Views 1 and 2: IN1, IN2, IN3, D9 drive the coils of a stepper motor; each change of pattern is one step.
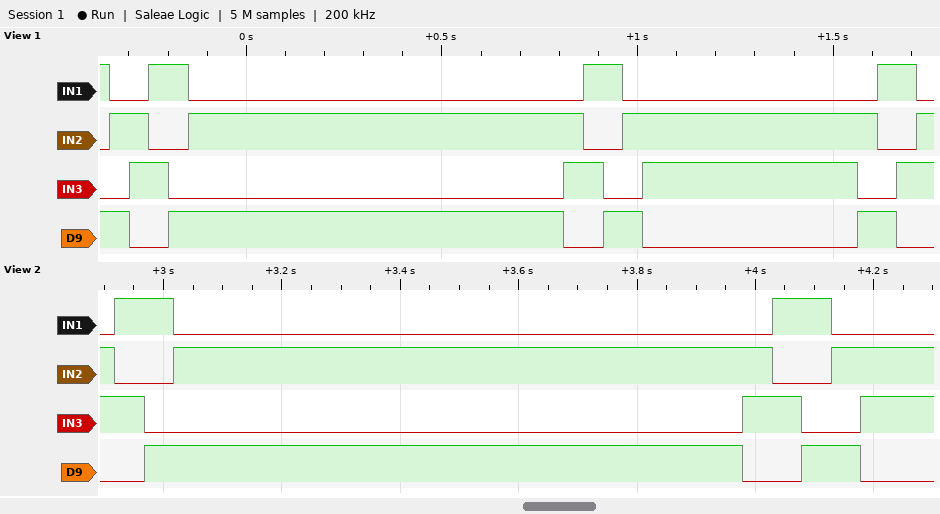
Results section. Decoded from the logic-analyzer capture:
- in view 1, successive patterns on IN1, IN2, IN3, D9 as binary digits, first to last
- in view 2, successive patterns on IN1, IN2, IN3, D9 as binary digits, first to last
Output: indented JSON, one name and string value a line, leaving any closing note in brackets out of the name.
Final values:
{
  "in view 1, successive patterns on IN1, IN2, IN3, D9 as binary digits, first to last": "1001 0101 0110 1010 1001 0101 0110 1010 1001 0101 0110 0101 1001 1010 0110",
  "in view 2, successive patterns on IN1, IN2, IN3, D9 as binary digits, first to last": "0110 1010 1001 0101 0110 1010 1001 0101 0110"
}
